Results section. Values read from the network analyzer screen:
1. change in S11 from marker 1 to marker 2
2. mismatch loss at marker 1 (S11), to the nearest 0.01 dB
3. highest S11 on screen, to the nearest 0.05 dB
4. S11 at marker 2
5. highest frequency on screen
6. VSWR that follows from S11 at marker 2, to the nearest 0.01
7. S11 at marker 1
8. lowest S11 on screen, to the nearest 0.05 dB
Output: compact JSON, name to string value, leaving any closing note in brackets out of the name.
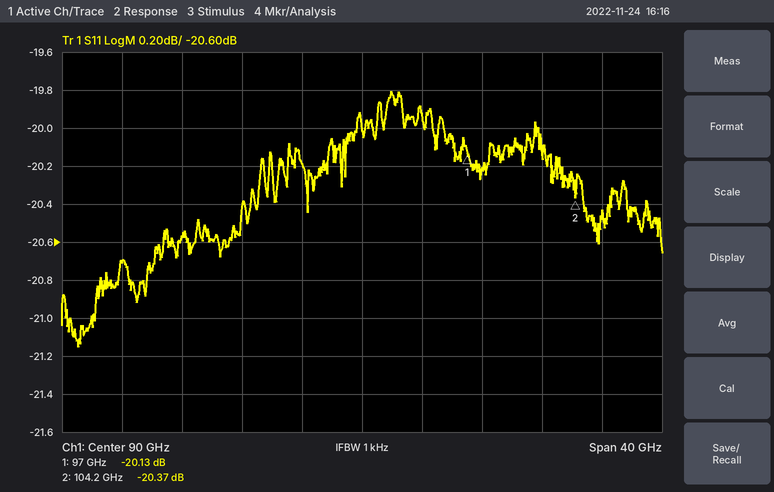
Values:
{"change in S11 from marker 1 to marker 2": "-0.24 dB", "mismatch loss at marker 1 (S11), to the nearest 0.01 dB": "0.04 dB", "highest S11 on screen, to the nearest 0.05 dB": "-19.80 dB", "S11 at marker 2": "-20.37 dB", "highest frequency on screen": "110 GHz", "VSWR that follows from S11 at marker 2, to the nearest 0.01": "1.21", "S11 at marker 1": "-20.13 dB", "lowest S11 on screen, to the nearest 0.05 dB": "-21.15 dB"}
